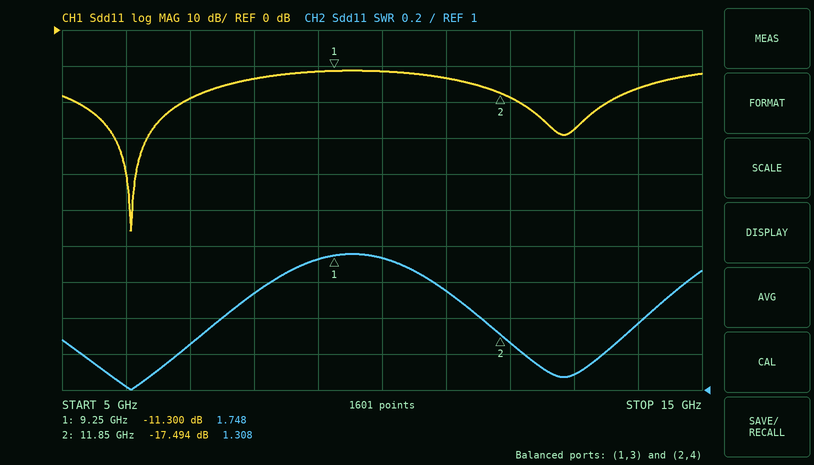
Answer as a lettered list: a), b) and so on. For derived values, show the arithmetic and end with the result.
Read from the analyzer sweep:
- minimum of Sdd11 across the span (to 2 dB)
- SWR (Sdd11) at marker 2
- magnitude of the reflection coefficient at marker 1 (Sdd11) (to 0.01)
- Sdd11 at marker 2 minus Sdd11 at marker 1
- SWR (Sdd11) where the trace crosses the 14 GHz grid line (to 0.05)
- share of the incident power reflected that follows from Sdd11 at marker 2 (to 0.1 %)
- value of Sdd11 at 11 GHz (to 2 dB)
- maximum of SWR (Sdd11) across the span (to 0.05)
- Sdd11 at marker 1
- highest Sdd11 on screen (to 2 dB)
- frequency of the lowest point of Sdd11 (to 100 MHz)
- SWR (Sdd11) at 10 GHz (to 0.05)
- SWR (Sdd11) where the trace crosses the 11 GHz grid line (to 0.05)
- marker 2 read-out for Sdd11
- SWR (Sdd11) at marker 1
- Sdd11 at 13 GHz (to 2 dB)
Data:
a) -56 dB
b) 1.308
c) 10^(-11.3/20) ≈ 0.27
d) -17.494 − (-11.3) = -6.194 dB
e) 1.35
f) 10^(-17.494/10) ≈ 1.8 %
g) -14 dB
h) 1.75
i) -11.300 dB
j) -12 dB
k) 6.1 GHz
l) 1.75
m) 1.55
n) -17.494 dB
o) 1.748
p) -28 dB
